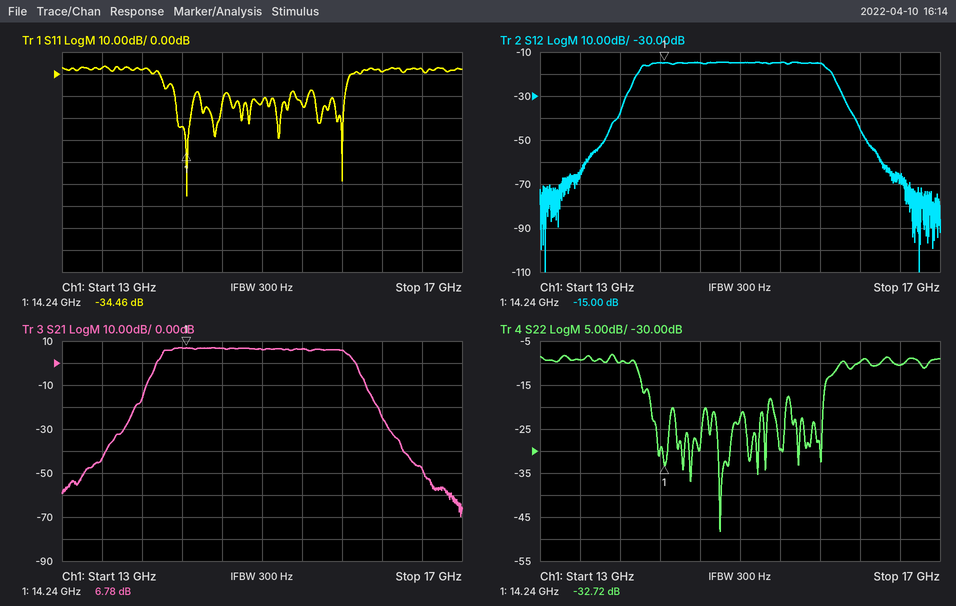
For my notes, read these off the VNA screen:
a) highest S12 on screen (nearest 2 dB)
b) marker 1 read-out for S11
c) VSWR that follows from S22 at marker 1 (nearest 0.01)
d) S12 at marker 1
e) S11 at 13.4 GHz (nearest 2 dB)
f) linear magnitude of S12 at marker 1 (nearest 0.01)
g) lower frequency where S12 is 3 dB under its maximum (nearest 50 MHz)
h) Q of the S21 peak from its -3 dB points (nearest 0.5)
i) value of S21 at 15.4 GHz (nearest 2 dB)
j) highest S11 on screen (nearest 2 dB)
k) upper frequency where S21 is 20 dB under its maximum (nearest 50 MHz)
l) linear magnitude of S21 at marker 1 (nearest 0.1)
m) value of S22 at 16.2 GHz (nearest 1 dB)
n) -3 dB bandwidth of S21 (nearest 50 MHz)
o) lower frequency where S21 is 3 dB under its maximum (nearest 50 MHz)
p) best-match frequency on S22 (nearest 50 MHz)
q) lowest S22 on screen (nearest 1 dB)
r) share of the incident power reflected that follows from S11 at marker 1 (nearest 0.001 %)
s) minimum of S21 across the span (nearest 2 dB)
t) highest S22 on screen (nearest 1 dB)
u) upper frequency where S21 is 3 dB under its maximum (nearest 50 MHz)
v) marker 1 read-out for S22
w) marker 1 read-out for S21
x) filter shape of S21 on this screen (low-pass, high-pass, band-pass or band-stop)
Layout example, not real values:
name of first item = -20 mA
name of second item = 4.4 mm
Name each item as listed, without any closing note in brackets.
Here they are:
highest S12 on screen = -14 dB
marker 1 read-out for S11 = -34.46 dB
VSWR that follows from S22 at marker 1 = 1.05
S12 at marker 1 = -15.00 dB
S11 at 13.4 GHz = 2 dB
linear magnitude of S12 at marker 1 = 0.18
lower frequency where S12 is 3 dB under its maximum = 14.00 GHz
Q of the S21 peak from its -3 dB points = 8.0
value of S21 at 15.4 GHz = 6 dB
highest S11 on screen = 4 dB
upper frequency where S21 is 20 dB under its maximum = 16.05 GHz
linear magnitude of S21 at marker 1 = 2.2
value of S22 at 16.2 GHz = -10 dB
-3 dB bandwidth of S21 = 1.85 GHz
lower frequency where S21 is 3 dB under its maximum = 14.00 GHz
best-match frequency on S22 = 14.80 GHz
lowest S22 on screen = -48 dB
share of the incident power reflected that follows from S11 at marker 1 = 0.036 %
minimum of S21 across the span = -70 dB
highest S22 on screen = -8 dB
upper frequency where S21 is 3 dB under its maximum = 15.85 GHz
marker 1 read-out for S22 = -32.72 dB
marker 1 read-out for S21 = 6.78 dB
filter shape of S21 on this screen = band-pass
